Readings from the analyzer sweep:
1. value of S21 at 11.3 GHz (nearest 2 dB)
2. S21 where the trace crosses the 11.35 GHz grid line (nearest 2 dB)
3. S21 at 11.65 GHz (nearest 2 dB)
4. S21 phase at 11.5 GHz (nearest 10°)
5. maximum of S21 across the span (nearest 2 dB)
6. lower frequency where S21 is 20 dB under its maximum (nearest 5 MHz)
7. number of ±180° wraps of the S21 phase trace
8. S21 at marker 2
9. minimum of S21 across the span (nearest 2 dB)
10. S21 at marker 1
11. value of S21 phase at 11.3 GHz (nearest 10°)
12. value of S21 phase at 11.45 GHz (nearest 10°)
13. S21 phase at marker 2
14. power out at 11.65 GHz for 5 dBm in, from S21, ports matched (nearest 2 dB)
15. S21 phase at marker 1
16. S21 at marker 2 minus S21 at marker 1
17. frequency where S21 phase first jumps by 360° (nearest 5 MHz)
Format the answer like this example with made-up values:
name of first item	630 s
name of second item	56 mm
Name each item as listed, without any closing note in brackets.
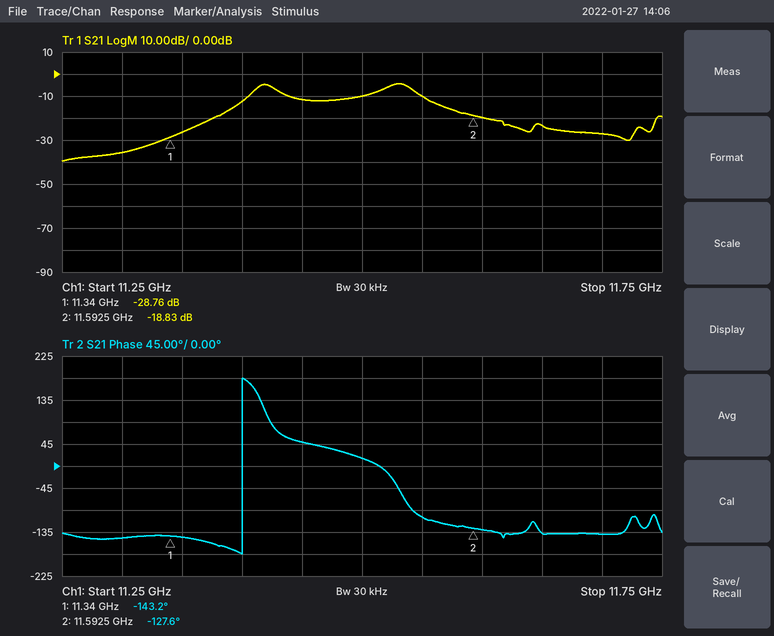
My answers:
value of S21 at 11.3 GHz	-36 dB
S21 where the trace crosses the 11.35 GHz grid line	-26 dB
S21 at 11.65 GHz	-24 dB
S21 phase at 11.5 GHz	20°
maximum of S21 across the span	-4 dB
lower frequency where S21 is 20 dB under its maximum	11.360 GHz
number of ±180° wraps of the S21 phase trace	1
S21 at marker 2	-18.83 dB
minimum of S21 across the span	-40 dB
S21 at marker 1	-28.76 dB
value of S21 phase at 11.3 GHz	-150°
value of S21 phase at 11.45 GHz	50°
S21 phase at marker 2	-127.6°
power out at 11.65 GHz for 5 dBm in, from S21, ports matched	-18 dBm
S21 phase at marker 1	-143.2°
S21 at marker 2 minus S21 at marker 1	9.93 dB
frequency where S21 phase first jumps by 360°	11.400 GHz
